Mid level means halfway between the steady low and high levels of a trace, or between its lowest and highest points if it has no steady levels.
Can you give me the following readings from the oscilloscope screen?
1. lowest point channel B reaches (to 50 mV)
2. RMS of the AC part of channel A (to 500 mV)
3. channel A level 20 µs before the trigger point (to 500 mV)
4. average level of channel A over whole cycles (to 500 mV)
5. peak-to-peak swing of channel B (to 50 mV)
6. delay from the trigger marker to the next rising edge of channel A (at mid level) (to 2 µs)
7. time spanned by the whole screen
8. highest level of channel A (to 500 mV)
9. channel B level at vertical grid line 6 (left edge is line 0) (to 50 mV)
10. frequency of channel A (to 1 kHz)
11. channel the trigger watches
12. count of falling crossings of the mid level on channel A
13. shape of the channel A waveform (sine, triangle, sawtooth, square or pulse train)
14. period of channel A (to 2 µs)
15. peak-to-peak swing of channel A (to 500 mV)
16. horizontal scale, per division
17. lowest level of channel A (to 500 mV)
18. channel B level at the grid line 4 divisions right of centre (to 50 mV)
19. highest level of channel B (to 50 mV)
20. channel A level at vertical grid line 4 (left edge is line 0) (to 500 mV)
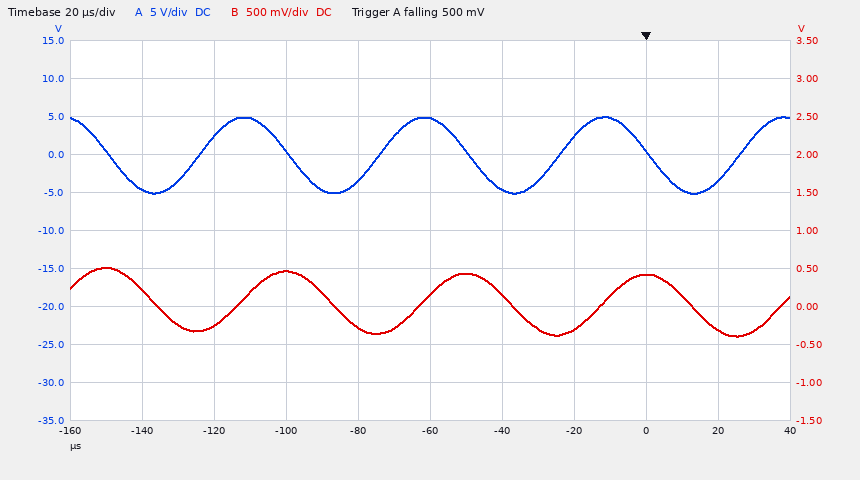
-400 mV
3.5 V
2.5 V
0.0 V
900 mV
26 µs
200 µs
5.0 V
150 mV
20 kHz
channel A
4
sine
50 µs
10.0 V
20 µs
-5.0 V
-300 mV
500 mV
-3.5 V
